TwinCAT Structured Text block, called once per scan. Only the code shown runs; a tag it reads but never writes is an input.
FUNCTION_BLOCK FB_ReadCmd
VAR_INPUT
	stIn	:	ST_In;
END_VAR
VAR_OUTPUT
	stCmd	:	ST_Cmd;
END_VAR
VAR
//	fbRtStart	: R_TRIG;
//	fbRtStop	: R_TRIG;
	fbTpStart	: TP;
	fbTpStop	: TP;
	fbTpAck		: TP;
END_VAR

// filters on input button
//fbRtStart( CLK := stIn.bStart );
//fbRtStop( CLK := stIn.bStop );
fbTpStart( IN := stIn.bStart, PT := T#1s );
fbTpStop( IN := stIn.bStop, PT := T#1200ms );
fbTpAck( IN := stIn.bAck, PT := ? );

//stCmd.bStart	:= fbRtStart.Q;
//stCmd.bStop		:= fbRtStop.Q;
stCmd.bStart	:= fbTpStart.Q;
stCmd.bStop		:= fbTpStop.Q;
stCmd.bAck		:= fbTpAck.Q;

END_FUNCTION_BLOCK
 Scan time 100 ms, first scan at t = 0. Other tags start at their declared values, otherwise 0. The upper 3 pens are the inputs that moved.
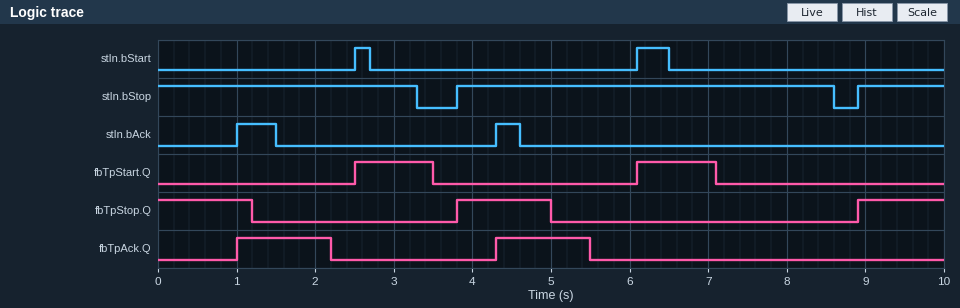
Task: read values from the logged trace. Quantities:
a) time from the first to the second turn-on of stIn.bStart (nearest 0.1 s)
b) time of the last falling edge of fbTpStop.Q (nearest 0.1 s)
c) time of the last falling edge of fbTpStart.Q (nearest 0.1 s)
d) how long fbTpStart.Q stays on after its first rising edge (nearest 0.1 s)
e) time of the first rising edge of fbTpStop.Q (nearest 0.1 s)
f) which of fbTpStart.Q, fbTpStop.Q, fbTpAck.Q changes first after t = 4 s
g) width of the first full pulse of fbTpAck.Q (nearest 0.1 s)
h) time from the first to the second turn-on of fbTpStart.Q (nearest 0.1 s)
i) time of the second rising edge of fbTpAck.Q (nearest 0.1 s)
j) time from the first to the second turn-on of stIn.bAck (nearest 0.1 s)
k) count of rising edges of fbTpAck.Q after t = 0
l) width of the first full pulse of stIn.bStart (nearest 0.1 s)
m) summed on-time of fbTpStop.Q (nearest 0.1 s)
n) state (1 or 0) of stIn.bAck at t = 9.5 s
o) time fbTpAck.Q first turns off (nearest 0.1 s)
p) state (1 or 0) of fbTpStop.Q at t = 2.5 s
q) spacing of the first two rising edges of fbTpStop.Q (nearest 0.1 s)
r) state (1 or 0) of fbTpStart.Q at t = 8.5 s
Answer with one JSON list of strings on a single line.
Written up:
["3.6 s", "5.0 s", "7.1 s", "1.0 s", "3.8 s", "fbTpAck.Q", "1.2 s", "3.6 s", "4.3 s", "3.3 s", "2", "0.2 s", "3.5 s", "0", "2.2 s", "0", "5.1 s", "0"]
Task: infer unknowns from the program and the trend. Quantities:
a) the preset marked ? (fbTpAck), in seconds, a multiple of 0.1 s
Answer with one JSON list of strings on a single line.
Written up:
["1.2 s"]
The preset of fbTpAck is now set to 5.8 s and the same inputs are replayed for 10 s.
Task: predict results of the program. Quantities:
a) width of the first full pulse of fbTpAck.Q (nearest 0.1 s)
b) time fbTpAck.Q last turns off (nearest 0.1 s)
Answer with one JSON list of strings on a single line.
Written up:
["5.8 s", "6.8 s"]
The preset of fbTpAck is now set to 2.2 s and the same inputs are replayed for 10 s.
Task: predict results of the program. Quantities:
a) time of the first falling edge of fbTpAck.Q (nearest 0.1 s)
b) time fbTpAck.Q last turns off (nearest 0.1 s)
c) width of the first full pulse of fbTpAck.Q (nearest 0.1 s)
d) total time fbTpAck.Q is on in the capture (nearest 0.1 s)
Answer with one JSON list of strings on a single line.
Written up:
["3.2 s", "6.5 s", "2.2 s", "4.4 s"]
